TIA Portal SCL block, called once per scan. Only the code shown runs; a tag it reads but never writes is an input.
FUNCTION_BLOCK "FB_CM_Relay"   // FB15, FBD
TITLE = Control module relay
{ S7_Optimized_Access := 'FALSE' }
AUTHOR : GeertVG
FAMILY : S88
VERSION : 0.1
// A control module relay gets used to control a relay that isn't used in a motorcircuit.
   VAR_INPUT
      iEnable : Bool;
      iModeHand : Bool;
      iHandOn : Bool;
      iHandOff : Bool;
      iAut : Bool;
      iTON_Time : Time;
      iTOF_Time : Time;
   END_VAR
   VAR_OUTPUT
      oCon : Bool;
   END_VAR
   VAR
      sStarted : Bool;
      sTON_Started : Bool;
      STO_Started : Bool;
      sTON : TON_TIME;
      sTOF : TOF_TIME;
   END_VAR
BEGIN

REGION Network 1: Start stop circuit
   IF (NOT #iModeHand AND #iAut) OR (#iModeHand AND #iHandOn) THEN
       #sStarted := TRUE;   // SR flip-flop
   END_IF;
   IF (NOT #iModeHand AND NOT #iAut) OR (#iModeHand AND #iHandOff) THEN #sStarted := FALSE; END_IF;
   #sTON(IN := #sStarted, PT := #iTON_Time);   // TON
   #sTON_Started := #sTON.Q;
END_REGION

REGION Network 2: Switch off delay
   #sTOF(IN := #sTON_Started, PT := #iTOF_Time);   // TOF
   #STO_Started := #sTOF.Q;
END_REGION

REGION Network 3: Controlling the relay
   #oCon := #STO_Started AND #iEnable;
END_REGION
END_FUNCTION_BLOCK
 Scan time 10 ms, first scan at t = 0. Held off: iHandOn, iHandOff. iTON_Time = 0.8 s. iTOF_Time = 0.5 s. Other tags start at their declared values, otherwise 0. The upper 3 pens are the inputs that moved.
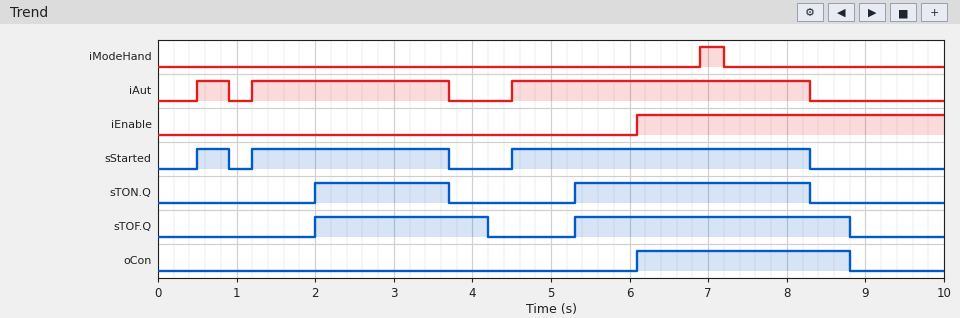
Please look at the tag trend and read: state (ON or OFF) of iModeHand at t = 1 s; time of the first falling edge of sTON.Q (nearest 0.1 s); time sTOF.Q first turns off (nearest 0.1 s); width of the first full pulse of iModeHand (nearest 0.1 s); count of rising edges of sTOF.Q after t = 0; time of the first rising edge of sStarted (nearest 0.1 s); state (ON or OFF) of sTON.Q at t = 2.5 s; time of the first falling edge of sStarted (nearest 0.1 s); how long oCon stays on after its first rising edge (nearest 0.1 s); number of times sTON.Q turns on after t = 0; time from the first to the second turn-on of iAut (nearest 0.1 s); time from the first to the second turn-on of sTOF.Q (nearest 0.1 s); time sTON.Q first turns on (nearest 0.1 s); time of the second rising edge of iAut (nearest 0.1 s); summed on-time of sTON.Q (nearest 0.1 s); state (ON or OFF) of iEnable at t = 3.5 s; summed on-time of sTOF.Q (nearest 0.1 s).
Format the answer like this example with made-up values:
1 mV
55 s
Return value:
OFF
3.7 s
4.2 s
0.3 s
2
0.5 s
ON
0.9 s
2.7 s
2
0.7 s
3.3 s
2.0 s
1.2 s
4.7 s
OFF
5.7 s
